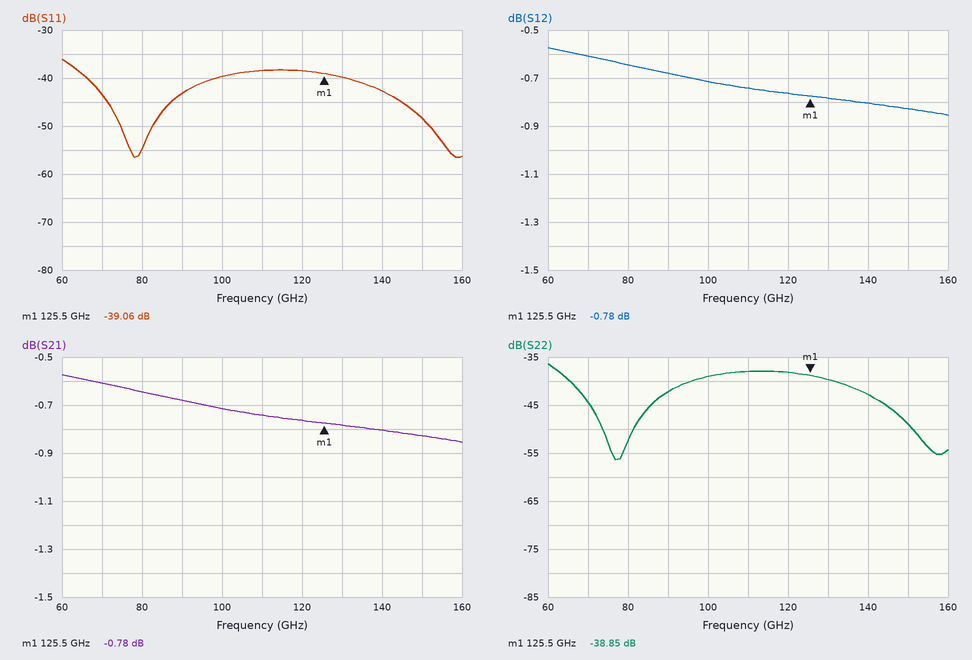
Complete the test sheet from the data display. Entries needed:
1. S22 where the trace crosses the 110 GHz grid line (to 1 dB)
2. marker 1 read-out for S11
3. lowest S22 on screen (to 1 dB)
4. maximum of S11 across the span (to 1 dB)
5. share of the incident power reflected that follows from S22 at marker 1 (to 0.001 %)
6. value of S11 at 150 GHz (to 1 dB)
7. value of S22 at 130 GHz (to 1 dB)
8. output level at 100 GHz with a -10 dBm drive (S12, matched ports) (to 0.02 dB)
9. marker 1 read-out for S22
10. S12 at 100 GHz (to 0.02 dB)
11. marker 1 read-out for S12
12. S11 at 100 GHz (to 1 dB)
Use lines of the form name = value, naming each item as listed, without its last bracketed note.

S22 where the trace crosses the 110 GHz grid line = -38 dB
marker 1 read-out for S11 = -39.06 dB
lowest S22 on screen = -56 dB
maximum of S11 across the span = -36 dB
share of the incident power reflected that follows from S22 at marker 1 = 0.013 %
value of S11 at 150 GHz = -48 dB
value of S22 at 130 GHz = -40 dB
output level at 100 GHz with a -10 dBm drive (S12, matched ports) = -10.72 dBm
marker 1 read-out for S22 = -38.85 dB
S12 at 100 GHz = -0.72 dB
marker 1 read-out for S12 = -0.78 dB
S11 at 100 GHz = -40 dB
